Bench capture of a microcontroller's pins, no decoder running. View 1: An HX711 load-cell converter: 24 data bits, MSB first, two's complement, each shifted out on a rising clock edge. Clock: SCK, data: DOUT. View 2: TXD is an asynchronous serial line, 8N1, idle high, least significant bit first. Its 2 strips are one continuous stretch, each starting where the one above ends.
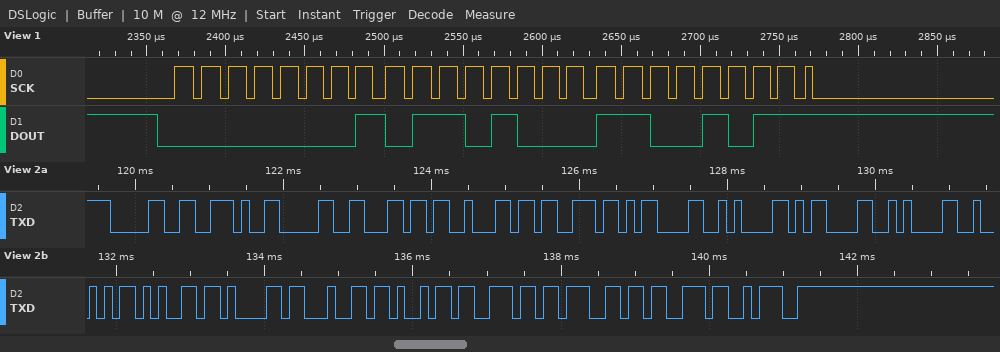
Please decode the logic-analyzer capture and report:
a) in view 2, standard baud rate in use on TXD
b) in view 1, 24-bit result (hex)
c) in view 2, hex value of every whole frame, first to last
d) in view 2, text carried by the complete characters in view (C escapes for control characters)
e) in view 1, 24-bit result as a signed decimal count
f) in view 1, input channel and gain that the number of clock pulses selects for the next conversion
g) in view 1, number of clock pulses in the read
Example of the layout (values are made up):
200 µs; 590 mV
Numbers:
9600 baud; 0x0168CB; 0x30 0x2E 0x30 0x6C 0x62 0x73 0x0D 0x0A 0x0D 0x0A 0x52 0x65 0x61 0x64 0x69 0x6E 0x67 0x73 0x3A; "0.0lbs\r\n\r\nReadings:"; 92363; channel A, gain 128; 25
